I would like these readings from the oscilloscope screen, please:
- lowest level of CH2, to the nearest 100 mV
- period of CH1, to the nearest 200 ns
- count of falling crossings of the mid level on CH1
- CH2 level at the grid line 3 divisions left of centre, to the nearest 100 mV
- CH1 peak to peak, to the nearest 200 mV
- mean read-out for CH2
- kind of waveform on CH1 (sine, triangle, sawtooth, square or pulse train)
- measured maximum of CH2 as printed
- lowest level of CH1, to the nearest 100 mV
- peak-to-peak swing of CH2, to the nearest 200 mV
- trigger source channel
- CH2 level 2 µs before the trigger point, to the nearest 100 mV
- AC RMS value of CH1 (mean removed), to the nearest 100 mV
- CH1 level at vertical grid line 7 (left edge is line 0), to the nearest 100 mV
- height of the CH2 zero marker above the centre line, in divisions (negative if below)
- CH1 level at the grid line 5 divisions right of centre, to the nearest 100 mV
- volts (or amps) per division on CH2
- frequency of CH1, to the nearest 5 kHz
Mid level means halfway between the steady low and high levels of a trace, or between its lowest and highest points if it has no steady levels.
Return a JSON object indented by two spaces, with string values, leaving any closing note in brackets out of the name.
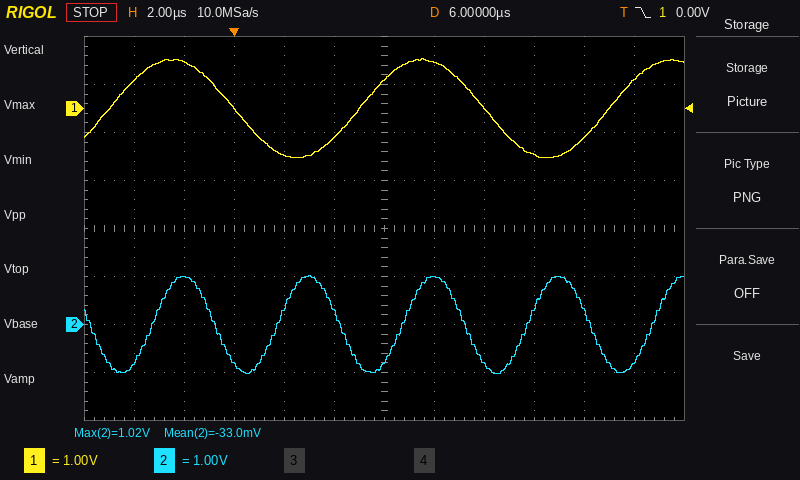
{
  "lowest level of CH2, to the nearest 100 mV": "-1.0 V",
  "period of CH1, to the nearest 200 ns": "10.0 µs",
  "count of falling crossings of the mid level on CH1": "2",
  "CH2 level at the grid line 3 divisions left of centre, to the nearest 100 mV": "-800 mV",
  "CH1 peak to peak, to the nearest 200 mV": "2.0 V",
  "mean read-out for CH2": "-33.0 mV",
  "kind of waveform on CH1": "sine",
  "measured maximum of CH2 as printed": "1.02 V",
  "lowest level of CH1, to the nearest 100 mV": "-1.0 V",
  "peak-to-peak swing of CH2, to the nearest 200 mV": "2.0 V",
  "trigger source channel": "CH1",
  "CH2 level 2 µs before the trigger point, to the nearest 100 mV": "1.0 V",
  "AC RMS value of CH1 (mean removed), to the nearest 100 mV": "700 mV",
  "CH1 level at vertical grid line 7 (left edge is line 0), to the nearest 100 mV": "1.0 V",
  "height of the CH2 zero marker above the centre line, in divisions": "-2.0 div",
  "CH1 level at the grid line 5 divisions right of centre, to the nearest 100 mV": "600 mV",
  "volts (or amps) per division on CH2": "1 V",
  "frequency of CH1, to the nearest 5 kHz": "100 kHz"
}
